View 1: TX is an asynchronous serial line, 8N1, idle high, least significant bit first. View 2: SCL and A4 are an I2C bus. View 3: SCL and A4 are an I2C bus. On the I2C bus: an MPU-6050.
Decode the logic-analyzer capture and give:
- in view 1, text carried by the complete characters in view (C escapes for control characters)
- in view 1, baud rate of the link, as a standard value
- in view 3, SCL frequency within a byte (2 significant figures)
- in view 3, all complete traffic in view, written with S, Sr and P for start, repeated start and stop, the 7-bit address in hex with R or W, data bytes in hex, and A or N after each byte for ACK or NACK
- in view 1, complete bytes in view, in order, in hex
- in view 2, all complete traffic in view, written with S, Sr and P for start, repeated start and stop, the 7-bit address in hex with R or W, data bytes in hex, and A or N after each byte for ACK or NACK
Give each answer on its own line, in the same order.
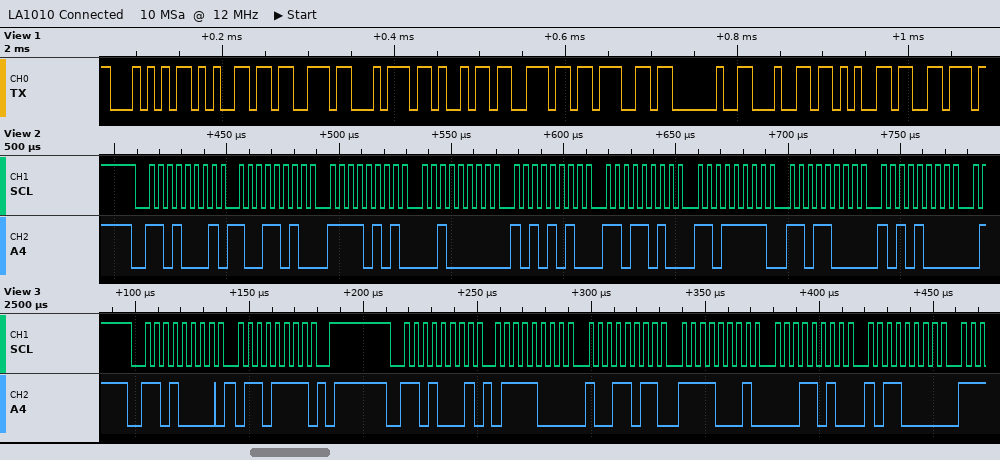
"Testing dev"
115200 baud
250 kHz
S 68W A 6F A P S 68R A 78 A 9B A F1 A 1A A B0 A
54 65 73 74 69 6E 67 20 64 65 76
S 68R A 9A A F5 A 20 A AA A DA A DF A D8 A A8 A
